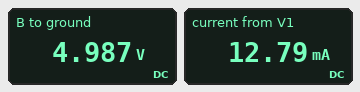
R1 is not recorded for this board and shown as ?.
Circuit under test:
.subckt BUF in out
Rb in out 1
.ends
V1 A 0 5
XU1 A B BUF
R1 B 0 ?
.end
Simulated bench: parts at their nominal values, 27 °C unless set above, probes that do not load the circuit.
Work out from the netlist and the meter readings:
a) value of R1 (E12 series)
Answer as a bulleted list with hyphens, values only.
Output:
- 390 Ω
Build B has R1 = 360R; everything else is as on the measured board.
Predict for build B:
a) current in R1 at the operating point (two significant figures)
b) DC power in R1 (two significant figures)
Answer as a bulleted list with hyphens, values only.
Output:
- 14 mA
- 69 mW
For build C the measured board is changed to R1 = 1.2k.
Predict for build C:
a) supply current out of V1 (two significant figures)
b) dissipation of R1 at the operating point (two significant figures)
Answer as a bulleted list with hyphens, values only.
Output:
- 4.2 mA
- 21 mW
